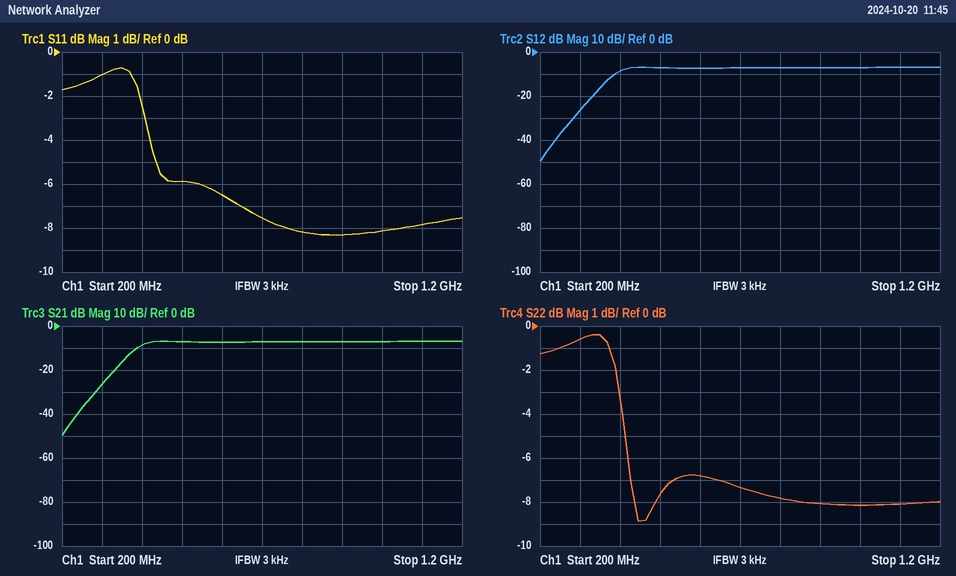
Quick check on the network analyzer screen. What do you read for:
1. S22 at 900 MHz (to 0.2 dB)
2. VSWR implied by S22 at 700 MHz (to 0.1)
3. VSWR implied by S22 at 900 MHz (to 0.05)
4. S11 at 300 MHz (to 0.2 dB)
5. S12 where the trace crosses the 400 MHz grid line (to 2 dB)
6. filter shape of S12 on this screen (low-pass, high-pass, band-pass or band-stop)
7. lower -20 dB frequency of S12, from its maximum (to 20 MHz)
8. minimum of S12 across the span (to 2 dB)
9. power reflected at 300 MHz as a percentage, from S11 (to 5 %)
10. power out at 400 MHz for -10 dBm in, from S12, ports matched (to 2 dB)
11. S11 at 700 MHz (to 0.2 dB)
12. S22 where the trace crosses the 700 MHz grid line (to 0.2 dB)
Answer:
-8.0 dB
2.5
2.30
-1.0 dB
-8 dB
high-pass
300 MHz
-50 dB
80 %
-18 dBm
-7.6 dB
-7.4 dB
